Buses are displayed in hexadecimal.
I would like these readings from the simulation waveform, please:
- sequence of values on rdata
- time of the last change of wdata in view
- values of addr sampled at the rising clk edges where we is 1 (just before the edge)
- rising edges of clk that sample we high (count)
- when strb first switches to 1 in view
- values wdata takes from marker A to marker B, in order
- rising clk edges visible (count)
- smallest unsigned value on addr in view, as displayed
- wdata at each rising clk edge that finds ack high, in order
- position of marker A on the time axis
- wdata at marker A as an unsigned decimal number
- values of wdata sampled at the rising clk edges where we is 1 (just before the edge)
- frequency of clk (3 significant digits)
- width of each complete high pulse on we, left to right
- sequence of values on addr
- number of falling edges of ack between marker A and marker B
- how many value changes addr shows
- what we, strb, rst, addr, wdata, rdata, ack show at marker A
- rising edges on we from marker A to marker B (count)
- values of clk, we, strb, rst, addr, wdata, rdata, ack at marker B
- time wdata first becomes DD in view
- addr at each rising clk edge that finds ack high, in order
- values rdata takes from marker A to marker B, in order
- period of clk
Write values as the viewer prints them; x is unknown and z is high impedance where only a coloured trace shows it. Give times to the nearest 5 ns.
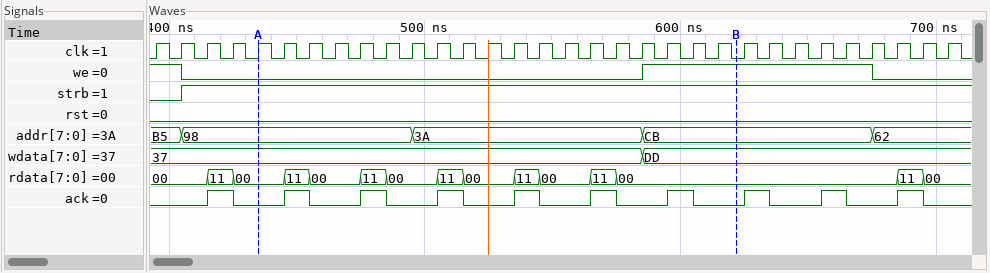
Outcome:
00, 11, 00, 11, 00, 11, 00, 11, 00, 11, 00, 11, 00, 11, 00
585 ns
B5, B5, CB, CB, CB, CB, CB, CB, CB, CB, CB
11
405 ns
37, DD
32
3A
37, 37, 37, 37, 37, 37, DD, DD, DD, DD
435 ns
55
37, 37, DD, DD, DD, DD, DD, DD, DD, DD, DD
100 MHz
90 ns
B5, 98, 3A, CB, 62
6
4
we=0, strb=1, rst=0, addr=98, wdata=37, rdata=00, ack=0
1
clk=0, we=1, strb=1, rst=0, addr=CB, wdata=DD, rdata=00, ack=0
585 ns
98, 98, 98, 3A, 3A, 3A, CB, CB, CB, 62
00, 11, 00, 11, 00, 11, 00, 11, 00, 11, 00
10 ns
